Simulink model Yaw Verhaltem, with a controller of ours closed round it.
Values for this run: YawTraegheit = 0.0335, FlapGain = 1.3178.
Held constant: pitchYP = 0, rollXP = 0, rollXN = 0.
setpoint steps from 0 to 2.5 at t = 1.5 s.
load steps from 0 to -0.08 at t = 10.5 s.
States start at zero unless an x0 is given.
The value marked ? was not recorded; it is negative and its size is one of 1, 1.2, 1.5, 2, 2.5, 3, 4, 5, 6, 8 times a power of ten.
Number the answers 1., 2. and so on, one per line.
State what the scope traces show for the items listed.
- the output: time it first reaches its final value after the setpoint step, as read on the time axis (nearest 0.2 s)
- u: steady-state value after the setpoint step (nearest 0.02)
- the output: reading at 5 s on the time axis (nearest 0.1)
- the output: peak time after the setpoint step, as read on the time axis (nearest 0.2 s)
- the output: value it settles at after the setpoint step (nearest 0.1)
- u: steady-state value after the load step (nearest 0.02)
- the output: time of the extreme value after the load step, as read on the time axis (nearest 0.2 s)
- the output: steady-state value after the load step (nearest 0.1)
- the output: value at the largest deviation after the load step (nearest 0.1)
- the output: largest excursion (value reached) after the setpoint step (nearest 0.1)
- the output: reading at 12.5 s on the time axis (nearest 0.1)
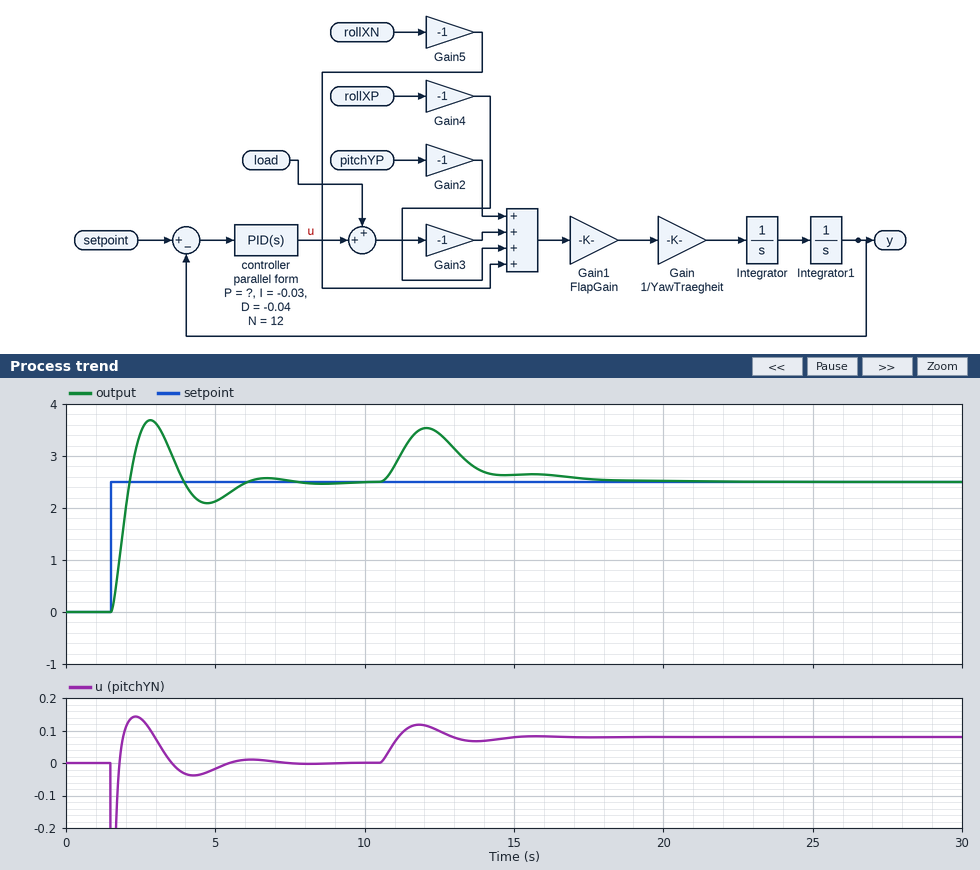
1. 2.2 s
2. 0.00
3. 2.1
4. 2.8 s
5. 2.5
6. 0.08
7. 12.0 s
8. 2.5
9. 3.5
10. 3.7
11. 3.4
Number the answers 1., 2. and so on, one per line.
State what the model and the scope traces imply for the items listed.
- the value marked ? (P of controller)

1. -0.08
